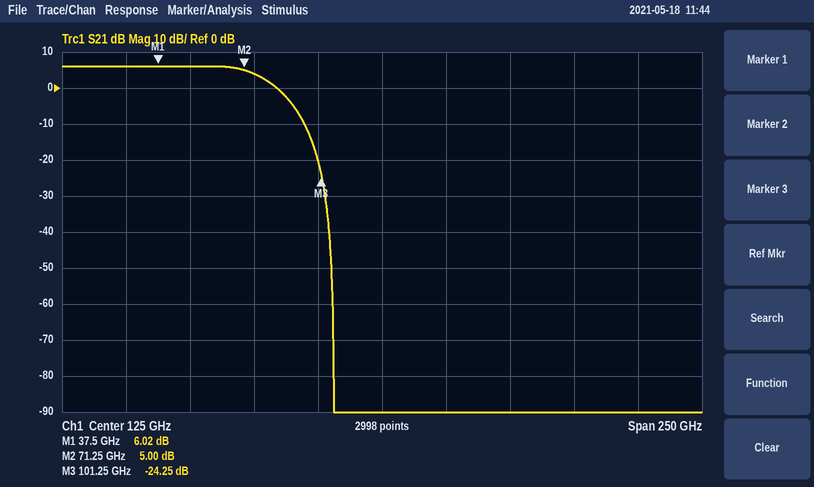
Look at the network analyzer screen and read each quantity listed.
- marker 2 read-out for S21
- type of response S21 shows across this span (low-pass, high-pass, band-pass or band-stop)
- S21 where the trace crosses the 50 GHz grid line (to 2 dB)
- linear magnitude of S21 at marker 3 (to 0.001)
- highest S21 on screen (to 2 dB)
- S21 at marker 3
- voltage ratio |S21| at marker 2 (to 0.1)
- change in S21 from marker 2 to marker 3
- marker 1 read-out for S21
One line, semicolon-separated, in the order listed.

5.00 dB; low-pass; 6 dB; 0.061; 6 dB; -24.25 dB; 1.8; -29.25 dB; 6.02 dB
